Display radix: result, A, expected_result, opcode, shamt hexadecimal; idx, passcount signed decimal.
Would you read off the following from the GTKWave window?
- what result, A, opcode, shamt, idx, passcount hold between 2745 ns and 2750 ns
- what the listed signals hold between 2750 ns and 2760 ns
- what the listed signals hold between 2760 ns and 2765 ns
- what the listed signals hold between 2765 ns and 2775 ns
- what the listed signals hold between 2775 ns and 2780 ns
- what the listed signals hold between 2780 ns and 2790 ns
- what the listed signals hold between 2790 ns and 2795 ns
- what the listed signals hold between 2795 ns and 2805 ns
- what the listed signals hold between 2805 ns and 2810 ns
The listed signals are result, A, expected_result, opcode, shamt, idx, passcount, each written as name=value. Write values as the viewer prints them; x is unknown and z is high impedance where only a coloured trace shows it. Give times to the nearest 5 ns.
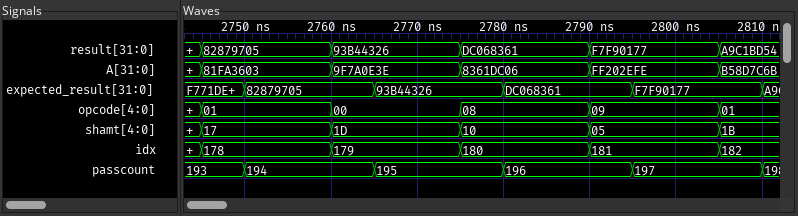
result=82879705, A=81FA3603, opcode=01, shamt=17, idx=178, passcount=193
result=82879705, A=81FA3603, expected_result=82879705, opcode=01, shamt=17, idx=178, passcount=194
result=93B44326, A=9F7A0E3E, expected_result=82879705, opcode=00, shamt=1D, idx=179, passcount=194
result=93B44326, A=9F7A0E3E, expected_result=93B44326, opcode=00, shamt=1D, idx=179, passcount=195
result=DC068361, A=8361DC06, expected_result=93B44326, opcode=08, shamt=10, idx=180, passcount=195
result=DC068361, A=8361DC06, expected_result=DC068361, opcode=08, shamt=10, idx=180, passcount=196
result=F7F90177, A=FF202EFE, expected_result=DC068361, opcode=09, shamt=05, idx=181, passcount=196
result=F7F90177, A=FF202EFE, expected_result=F7F90177, opcode=09, shamt=05, idx=181, passcount=197
result=A9C1BD54, A=B58D7C6B, expected_result=F7F90177, opcode=01, shamt=1B, idx=182, passcount=197
